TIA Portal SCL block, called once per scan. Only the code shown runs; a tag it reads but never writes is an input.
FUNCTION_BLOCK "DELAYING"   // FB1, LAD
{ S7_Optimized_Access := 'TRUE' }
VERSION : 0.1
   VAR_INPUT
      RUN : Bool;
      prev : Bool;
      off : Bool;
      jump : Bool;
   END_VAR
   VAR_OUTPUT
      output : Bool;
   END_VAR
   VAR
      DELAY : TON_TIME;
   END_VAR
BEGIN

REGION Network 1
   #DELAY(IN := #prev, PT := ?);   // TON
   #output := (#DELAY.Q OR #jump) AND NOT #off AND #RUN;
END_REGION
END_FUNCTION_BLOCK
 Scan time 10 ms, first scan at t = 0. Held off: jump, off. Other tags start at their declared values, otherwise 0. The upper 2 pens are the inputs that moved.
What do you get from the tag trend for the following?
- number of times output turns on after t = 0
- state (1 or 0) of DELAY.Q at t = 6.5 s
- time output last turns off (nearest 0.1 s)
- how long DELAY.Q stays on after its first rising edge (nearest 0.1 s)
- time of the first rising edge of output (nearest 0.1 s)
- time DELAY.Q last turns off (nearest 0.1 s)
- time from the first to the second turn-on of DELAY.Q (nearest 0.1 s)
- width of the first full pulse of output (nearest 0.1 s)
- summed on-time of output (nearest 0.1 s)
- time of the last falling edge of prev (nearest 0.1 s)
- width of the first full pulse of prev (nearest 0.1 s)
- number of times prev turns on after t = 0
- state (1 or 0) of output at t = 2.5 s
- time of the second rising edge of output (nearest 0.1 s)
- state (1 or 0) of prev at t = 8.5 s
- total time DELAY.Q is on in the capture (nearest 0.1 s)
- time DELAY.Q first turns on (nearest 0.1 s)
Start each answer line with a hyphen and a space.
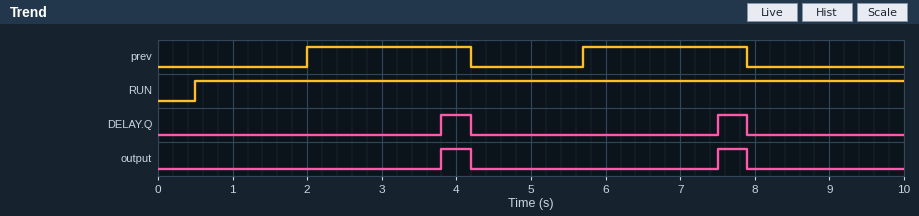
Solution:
- 2
- 0
- 7.9 s
- 0.4 s
- 3.8 s
- 7.9 s
- 3.7 s
- 0.4 s
- 0.8 s
- 7.9 s
- 2.2 s
- 2
- 0
- 7.5 s
- 0
- 0.8 s
- 3.8 s
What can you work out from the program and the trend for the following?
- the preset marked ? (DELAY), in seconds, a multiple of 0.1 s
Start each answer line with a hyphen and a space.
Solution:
- 1.8 s
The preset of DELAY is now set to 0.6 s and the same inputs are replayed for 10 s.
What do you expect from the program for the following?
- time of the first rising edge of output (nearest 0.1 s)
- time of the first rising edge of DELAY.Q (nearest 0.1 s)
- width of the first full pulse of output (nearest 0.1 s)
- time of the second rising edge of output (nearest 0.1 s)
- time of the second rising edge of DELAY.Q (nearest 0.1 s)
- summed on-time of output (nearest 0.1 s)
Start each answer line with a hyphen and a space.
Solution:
- 2.6 s
- 2.6 s
- 1.6 s
- 6.3 s
- 6.3 s
- 3.2 s
